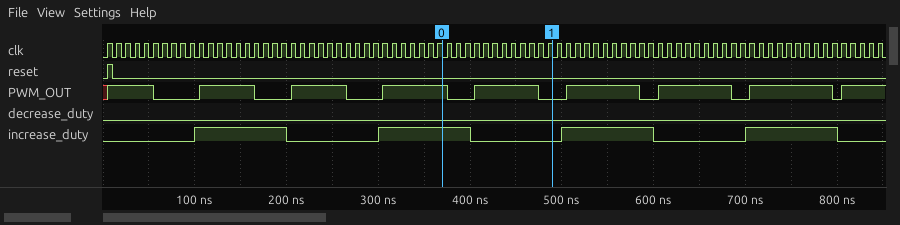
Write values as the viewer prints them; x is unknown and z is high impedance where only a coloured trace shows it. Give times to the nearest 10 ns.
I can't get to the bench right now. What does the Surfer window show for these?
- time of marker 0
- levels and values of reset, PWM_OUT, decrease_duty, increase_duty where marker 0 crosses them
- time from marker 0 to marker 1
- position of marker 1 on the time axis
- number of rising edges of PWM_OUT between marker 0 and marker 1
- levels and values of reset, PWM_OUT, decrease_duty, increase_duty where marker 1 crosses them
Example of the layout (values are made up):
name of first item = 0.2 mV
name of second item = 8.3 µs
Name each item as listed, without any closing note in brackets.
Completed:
time of marker 0 = 370 ns
levels and values of reset, PWM_OUT, decrease_duty, increase_duty where marker 0 crosses them = reset=0, PWM_OUT=1, decrease_duty=0, increase_duty=1
time from marker 0 to marker 1 = 120 ns
position of marker 1 on the time axis = 490 ns
number of rising edges of PWM_OUT between marker 0 and marker 1 = 1
levels and values of reset, PWM_OUT, decrease_duty, increase_duty where marker 1 crosses them = reset=0, PWM_OUT=0, decrease_duty=0, increase_duty=0
